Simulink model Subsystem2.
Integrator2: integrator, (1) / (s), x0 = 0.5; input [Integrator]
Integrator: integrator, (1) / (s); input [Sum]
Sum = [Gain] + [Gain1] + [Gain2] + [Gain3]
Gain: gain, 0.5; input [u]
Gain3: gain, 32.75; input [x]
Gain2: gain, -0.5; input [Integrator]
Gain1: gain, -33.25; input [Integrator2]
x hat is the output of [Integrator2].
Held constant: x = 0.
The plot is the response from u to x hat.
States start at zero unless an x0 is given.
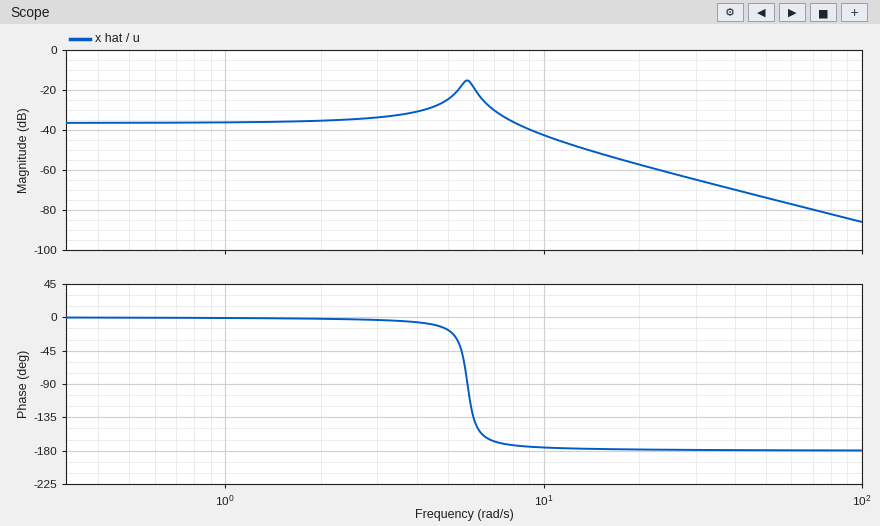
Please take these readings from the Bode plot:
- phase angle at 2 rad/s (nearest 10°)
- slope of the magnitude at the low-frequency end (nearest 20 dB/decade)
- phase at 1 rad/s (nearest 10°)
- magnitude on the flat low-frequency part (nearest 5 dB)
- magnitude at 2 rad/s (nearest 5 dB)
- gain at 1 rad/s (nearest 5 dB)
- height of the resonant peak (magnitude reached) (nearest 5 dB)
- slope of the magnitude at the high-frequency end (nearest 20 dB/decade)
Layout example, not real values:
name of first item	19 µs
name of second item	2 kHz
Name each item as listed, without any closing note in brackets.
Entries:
phase angle at 2 rad/s	0°
slope of the magnitude at the low-frequency end	0 dB/decade
phase at 1 rad/s	0°
magnitude on the flat low-frequency part	-35 dB
magnitude at 2 rad/s	-35 dB
gain at 1 rad/s	-35 dB
height of the resonant peak (magnitude reached)	-15 dB
slope of the magnitude at the high-frequency end	-40 dB/decade
